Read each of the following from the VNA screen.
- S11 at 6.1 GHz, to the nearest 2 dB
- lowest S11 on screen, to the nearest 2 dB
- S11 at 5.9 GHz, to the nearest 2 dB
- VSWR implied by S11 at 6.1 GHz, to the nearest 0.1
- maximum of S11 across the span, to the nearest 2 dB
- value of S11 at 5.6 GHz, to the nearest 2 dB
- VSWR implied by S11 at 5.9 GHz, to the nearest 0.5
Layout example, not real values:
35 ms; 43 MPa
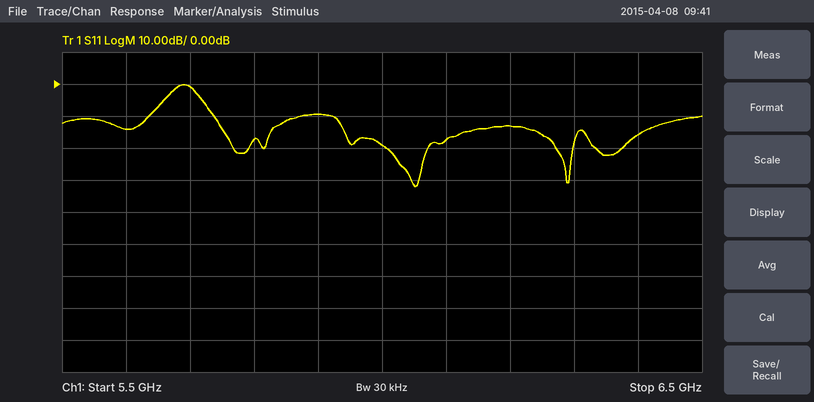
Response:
-18 dB; -32 dB; -10 dB; 1.3; 0 dB; -14 dB; 2.0
